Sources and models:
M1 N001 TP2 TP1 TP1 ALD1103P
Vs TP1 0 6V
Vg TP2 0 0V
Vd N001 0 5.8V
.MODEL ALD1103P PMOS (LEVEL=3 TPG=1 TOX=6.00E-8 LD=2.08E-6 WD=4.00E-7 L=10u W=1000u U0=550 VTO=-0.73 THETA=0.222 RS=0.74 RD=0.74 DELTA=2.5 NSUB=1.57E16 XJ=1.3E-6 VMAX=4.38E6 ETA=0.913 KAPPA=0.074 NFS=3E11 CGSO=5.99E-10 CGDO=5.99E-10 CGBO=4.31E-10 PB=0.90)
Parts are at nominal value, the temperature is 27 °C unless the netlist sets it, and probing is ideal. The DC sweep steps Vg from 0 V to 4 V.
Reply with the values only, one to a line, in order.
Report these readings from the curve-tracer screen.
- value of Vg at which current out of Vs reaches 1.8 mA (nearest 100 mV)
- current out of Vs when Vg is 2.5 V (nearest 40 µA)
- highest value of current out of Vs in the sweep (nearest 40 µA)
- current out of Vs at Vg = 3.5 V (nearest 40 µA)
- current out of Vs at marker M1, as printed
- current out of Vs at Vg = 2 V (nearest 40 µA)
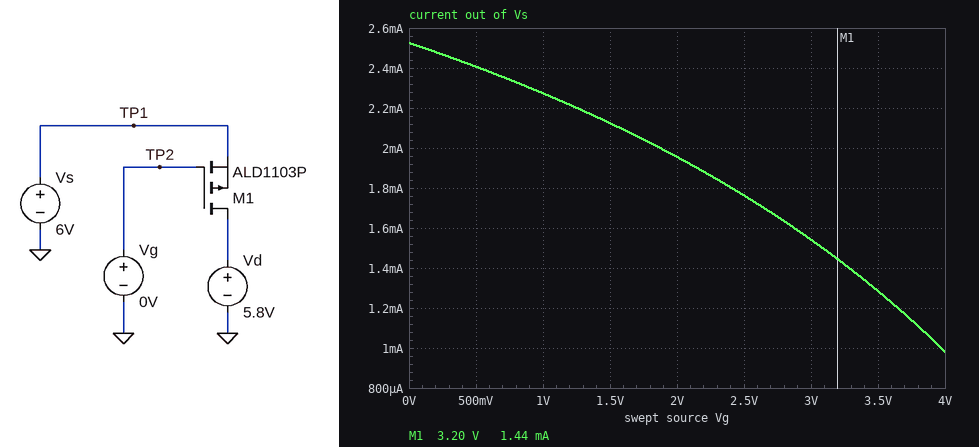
2.4 V
1.76 mA
2.52 mA
1.28 mA
1.44 mA
1.96 mA
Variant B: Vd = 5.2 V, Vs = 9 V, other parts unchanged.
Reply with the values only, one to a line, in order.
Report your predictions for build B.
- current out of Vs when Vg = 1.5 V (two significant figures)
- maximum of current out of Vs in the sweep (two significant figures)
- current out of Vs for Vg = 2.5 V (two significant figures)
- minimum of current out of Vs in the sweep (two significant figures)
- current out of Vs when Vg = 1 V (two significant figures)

34 mA
41 mA
29 mA
19 mA
37 mA
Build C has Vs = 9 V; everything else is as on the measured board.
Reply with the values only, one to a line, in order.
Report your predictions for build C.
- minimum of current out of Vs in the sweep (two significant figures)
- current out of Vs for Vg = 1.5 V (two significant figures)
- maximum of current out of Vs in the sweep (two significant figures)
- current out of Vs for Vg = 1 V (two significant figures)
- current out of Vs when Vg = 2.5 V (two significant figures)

19 mA
32 mA
37 mA
34 mA
27 mA
